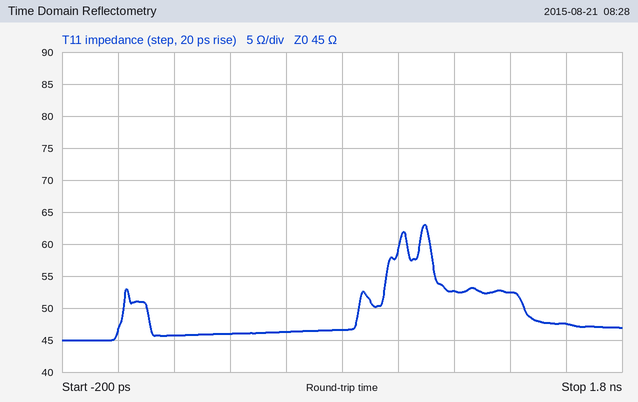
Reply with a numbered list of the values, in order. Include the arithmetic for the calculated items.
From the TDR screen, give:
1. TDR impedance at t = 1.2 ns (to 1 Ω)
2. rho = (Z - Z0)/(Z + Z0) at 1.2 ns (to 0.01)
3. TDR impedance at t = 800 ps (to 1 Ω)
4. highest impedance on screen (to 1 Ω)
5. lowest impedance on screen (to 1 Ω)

1. 53 Ω
2. (53 − 45)/(53 + 45) ≈ +0.08
3. 47 Ω
4. 63 Ω
5. 45 Ω
